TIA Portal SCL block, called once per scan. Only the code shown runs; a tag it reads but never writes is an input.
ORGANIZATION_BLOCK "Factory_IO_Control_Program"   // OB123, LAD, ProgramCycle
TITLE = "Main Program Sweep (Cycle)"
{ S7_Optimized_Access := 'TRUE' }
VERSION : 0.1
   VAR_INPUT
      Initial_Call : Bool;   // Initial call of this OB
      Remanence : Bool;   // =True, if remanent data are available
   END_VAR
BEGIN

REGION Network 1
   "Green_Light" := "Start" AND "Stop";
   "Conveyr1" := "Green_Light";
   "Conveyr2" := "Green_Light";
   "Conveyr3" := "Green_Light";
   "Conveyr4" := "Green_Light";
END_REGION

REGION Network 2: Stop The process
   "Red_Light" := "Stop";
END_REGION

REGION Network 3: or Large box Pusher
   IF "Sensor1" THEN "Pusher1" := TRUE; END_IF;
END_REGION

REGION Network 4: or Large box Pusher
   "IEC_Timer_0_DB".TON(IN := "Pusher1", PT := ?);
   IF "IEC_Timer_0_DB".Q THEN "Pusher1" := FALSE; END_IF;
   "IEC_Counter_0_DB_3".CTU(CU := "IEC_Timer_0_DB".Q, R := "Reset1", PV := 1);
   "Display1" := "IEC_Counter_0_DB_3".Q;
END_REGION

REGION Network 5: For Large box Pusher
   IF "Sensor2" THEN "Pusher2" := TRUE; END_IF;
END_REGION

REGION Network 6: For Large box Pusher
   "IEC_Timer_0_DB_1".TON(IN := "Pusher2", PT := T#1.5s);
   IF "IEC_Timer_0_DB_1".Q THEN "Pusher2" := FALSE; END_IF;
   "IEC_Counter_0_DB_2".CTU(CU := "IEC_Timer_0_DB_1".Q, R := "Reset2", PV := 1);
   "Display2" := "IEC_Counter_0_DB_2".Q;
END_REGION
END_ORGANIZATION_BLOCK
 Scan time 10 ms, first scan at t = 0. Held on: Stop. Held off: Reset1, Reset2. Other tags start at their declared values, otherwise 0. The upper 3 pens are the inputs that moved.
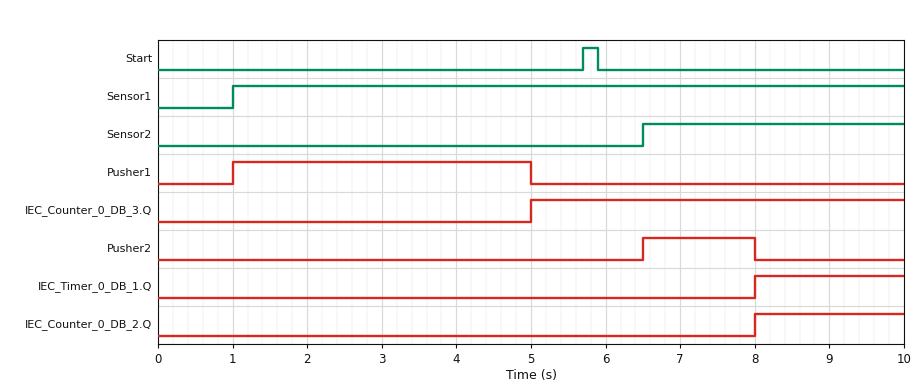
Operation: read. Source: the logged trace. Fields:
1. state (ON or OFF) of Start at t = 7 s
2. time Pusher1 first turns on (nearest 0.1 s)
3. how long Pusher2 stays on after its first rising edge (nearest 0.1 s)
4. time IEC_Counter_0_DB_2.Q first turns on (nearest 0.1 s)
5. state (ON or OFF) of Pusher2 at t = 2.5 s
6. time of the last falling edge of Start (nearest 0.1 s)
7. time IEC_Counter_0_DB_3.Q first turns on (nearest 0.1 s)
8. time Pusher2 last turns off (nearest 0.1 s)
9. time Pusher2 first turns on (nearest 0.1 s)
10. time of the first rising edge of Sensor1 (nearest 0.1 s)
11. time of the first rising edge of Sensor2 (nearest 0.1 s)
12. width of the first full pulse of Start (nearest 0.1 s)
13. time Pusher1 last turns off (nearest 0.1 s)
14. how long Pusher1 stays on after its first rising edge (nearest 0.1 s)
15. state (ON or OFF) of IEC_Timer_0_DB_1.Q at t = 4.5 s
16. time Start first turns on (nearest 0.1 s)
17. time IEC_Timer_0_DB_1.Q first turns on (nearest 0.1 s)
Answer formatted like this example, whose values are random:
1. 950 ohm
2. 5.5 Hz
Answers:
1. OFF
2. 1.0 s
3. 1.5 s
4. 8.0 s
5. OFF
6. 5.9 s
7. 5.0 s
8. 8.0 s
9. 6.5 s
10. 1.0 s
11. 6.5 s
12. 0.2 s
13. 5.0 s
14. 4.0 s
15. OFF
16. 5.7 s
17. 8.0 s
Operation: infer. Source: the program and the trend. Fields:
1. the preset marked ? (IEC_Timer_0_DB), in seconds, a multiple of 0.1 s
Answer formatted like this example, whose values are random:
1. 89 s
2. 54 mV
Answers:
1. 4.0 s
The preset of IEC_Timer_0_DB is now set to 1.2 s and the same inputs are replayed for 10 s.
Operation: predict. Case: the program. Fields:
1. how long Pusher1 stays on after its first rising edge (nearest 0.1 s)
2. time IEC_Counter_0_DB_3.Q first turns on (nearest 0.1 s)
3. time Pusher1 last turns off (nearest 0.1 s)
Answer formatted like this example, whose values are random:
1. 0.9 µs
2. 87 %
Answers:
1. 1.2 s
2. 2.2 s
3. 2.2 s
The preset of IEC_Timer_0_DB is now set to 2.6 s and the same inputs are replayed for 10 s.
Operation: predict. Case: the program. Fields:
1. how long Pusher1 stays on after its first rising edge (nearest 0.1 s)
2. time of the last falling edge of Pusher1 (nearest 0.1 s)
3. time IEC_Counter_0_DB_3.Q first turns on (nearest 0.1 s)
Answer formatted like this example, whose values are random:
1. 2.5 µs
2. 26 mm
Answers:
1. 2.6 s
2. 3.6 s
3. 3.6 s
